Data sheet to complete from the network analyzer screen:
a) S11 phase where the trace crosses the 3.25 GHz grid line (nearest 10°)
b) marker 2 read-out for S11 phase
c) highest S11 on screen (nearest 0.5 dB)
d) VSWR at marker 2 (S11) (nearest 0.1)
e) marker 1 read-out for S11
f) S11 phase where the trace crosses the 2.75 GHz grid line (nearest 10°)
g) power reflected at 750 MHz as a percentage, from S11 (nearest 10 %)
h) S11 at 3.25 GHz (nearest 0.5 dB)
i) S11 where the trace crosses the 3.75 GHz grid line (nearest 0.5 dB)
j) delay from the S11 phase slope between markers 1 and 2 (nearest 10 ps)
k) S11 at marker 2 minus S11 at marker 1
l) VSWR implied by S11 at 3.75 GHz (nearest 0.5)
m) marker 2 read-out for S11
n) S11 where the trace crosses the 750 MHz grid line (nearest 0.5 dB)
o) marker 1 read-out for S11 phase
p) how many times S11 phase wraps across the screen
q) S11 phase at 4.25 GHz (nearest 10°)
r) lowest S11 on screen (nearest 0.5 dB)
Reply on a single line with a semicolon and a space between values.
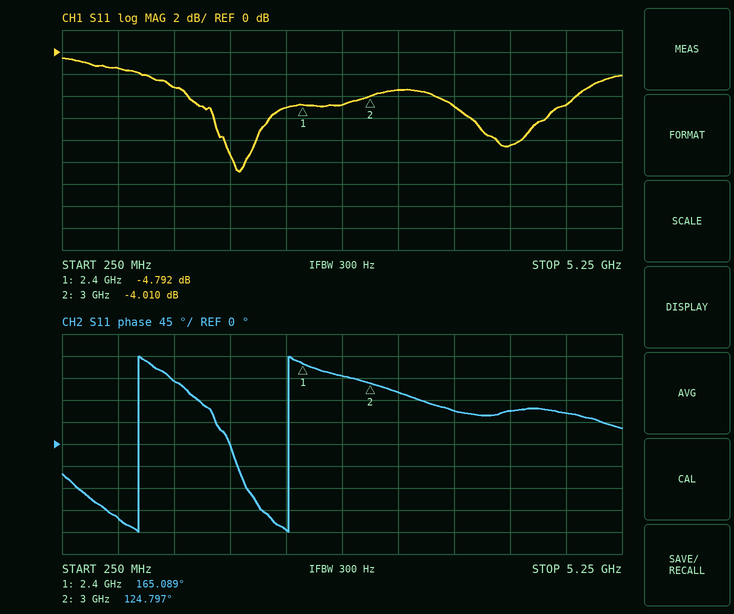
110°; 124.797°; -0.5 dB; 4.4; -4.792 dB; 140°; 70 %; -3.5 dB; -5.0 dB; 190 ps; 0.782 dB; 3.5; -4.010 dB; -1.5 dB; 165.089°; 2; 70°; -11.0 dB
